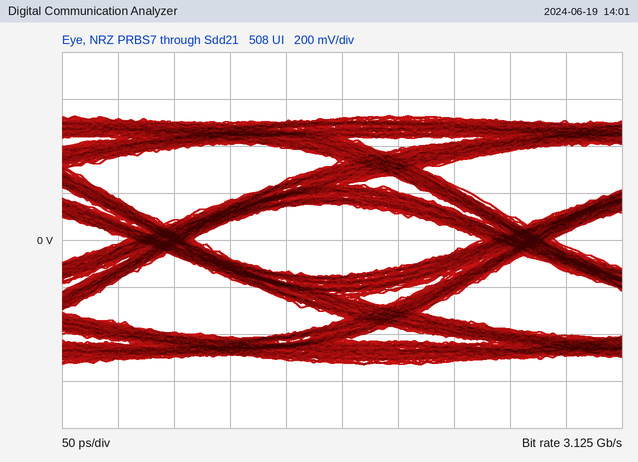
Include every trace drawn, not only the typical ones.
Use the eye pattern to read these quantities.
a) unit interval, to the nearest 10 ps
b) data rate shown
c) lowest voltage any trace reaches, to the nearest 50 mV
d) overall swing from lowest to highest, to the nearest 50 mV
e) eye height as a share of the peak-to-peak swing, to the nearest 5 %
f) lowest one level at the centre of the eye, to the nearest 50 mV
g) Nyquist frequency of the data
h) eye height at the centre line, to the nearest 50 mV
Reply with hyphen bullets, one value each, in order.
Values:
- 320 ps
- 3.125 Gb/s
- -550 mV
- 1.05 V
- 30 %
- 150 mV
- 1.5625 GHz
- 300 mV
